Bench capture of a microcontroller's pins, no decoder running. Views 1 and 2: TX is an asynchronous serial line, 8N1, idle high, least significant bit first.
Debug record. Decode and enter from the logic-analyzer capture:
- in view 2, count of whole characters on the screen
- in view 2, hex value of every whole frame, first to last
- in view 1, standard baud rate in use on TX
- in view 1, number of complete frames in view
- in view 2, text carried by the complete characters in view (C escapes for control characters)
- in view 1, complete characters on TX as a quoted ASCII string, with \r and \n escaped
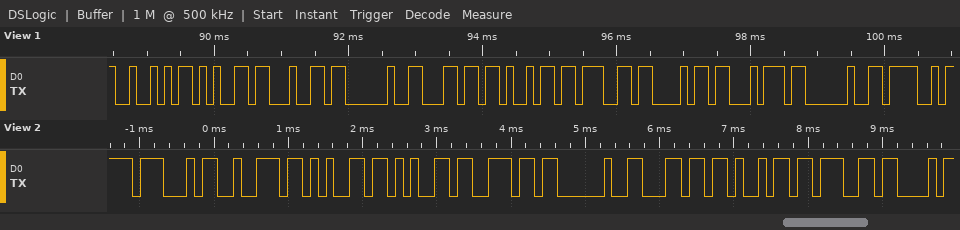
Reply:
9
47 72 65 65 6E 20 6C 69 67
9600 baud
11
"Green lig"
"Red light O"
